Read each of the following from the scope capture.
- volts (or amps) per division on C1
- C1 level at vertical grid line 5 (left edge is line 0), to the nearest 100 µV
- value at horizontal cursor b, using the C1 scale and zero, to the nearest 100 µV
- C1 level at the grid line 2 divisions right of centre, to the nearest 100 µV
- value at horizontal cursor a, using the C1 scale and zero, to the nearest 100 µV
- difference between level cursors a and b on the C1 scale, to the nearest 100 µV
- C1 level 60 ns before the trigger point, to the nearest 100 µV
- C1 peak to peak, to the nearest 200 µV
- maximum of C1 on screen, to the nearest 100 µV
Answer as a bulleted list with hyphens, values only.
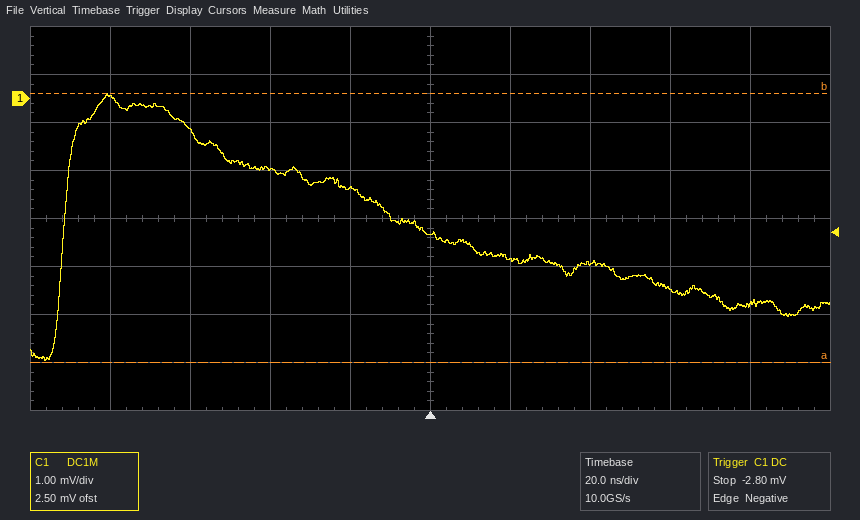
- 1 mV
- -2.8 mV
- 100 µV
- -3.4 mV
- -5.5 mV
- 5.6 mV
- -700 µV
- 5.6 mV
- 100 µV
